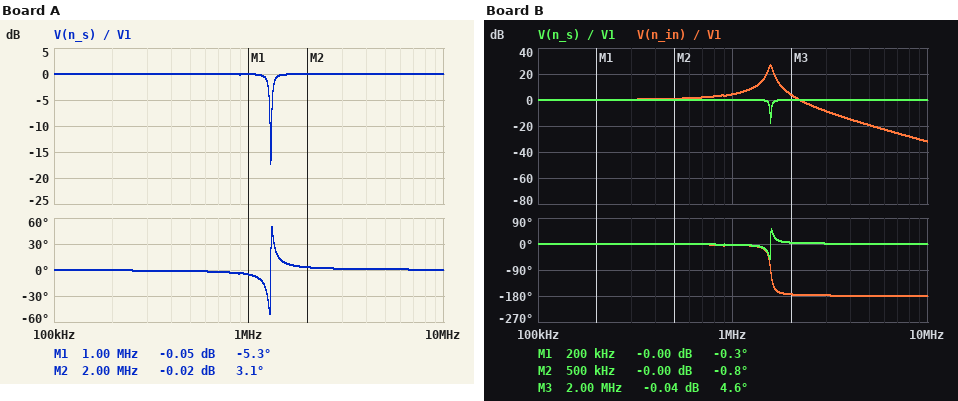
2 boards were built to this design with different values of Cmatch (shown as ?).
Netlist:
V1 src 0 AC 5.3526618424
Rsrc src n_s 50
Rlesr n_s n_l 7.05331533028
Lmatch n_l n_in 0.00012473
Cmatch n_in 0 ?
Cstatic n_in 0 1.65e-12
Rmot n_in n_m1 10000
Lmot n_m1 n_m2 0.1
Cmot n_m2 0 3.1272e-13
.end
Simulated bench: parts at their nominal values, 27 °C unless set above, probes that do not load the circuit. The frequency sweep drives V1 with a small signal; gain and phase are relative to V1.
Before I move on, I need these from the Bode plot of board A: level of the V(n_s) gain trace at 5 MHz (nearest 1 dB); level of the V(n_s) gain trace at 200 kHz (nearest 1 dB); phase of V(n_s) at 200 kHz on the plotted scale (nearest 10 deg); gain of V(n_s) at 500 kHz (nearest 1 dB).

0 dB
0 dB
0 deg
0 dB
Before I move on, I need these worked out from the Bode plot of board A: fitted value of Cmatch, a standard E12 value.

120 pF
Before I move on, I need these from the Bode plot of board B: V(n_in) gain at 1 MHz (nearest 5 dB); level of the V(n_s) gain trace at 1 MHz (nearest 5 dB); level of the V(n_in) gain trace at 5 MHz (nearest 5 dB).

5 dB
0 dB
-20 dB
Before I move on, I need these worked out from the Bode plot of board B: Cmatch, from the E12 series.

82 pF
